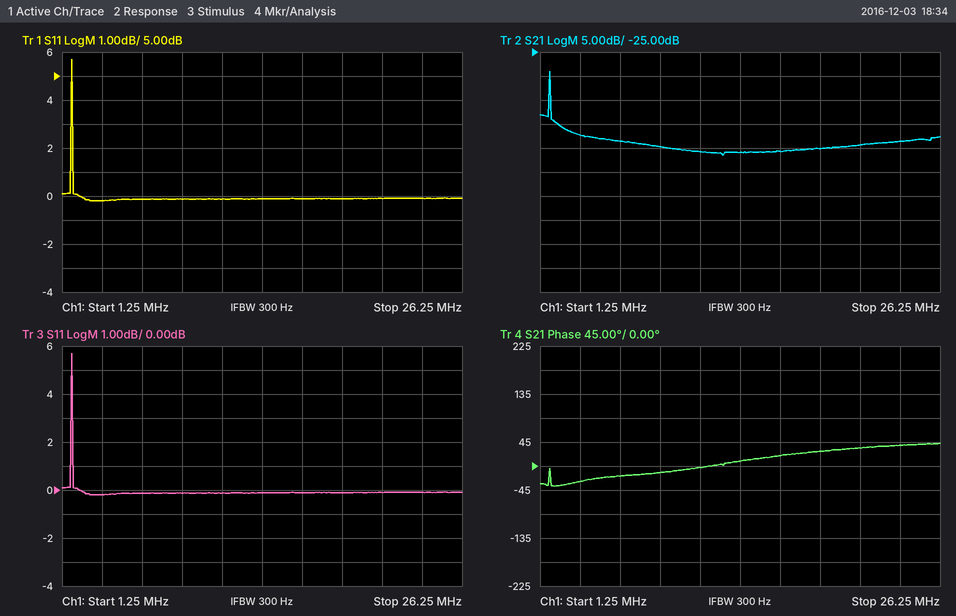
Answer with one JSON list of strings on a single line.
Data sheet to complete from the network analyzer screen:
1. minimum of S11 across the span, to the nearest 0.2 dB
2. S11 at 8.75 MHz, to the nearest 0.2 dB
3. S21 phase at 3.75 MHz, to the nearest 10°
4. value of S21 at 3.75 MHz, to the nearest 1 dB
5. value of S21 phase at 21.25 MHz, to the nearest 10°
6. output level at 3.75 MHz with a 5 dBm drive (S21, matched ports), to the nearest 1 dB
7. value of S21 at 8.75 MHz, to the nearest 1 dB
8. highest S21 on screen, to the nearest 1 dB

["-0.2 dB", "-0.2 dB", "-30°", "-42 dB", "30°", "-37 dBm", "-45 dB", "-29 dB"]
